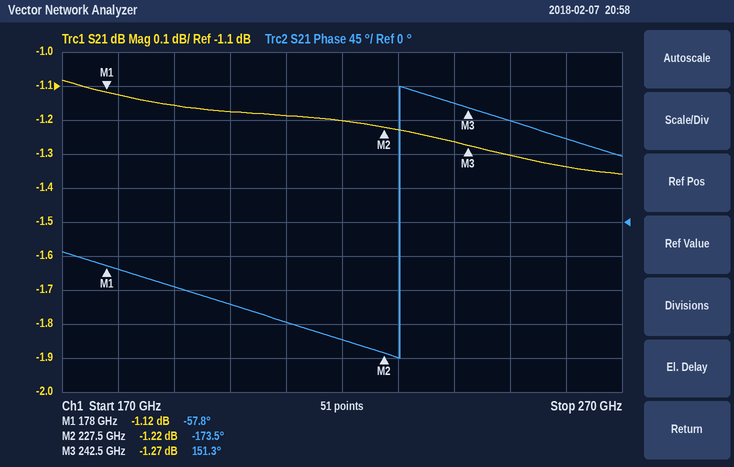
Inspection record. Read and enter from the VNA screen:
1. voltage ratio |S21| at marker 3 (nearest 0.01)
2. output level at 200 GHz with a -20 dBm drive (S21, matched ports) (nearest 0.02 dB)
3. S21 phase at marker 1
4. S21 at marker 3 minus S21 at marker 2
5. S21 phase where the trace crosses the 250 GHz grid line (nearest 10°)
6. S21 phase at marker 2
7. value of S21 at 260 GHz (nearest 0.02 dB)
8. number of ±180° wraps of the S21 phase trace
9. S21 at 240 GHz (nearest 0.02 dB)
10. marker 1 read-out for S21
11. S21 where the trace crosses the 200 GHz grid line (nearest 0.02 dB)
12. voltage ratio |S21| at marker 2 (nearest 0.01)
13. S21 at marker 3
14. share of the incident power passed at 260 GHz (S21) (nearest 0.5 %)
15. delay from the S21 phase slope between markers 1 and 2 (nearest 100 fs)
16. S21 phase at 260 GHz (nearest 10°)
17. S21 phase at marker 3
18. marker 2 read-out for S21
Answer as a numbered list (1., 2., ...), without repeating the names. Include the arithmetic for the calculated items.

1. 10^(-1.27/20) ≈ 0.86
2. -20 dBm + (-1.18 dB) = -21.18 dBm
3. -57.8°
4. -1.27 − (-1.22) = -0.05 dB
5. 130°
6. -173.5°
7. -1.34 dB
8. 1
9. -1.26 dB
10. -1.12 dB
11. -1.18 dB
12. 10^(-1.22/20) ≈ 0.87
13. -1.27 dB
14. 10^(-1.34/10) ≈ 73.5 %
15. −(-173.5° − (-57.8°))/(360° × 49.5 GHz) ≈ 6.5 ps
16. 110°
17. 151.3°
18. -1.22 dB
